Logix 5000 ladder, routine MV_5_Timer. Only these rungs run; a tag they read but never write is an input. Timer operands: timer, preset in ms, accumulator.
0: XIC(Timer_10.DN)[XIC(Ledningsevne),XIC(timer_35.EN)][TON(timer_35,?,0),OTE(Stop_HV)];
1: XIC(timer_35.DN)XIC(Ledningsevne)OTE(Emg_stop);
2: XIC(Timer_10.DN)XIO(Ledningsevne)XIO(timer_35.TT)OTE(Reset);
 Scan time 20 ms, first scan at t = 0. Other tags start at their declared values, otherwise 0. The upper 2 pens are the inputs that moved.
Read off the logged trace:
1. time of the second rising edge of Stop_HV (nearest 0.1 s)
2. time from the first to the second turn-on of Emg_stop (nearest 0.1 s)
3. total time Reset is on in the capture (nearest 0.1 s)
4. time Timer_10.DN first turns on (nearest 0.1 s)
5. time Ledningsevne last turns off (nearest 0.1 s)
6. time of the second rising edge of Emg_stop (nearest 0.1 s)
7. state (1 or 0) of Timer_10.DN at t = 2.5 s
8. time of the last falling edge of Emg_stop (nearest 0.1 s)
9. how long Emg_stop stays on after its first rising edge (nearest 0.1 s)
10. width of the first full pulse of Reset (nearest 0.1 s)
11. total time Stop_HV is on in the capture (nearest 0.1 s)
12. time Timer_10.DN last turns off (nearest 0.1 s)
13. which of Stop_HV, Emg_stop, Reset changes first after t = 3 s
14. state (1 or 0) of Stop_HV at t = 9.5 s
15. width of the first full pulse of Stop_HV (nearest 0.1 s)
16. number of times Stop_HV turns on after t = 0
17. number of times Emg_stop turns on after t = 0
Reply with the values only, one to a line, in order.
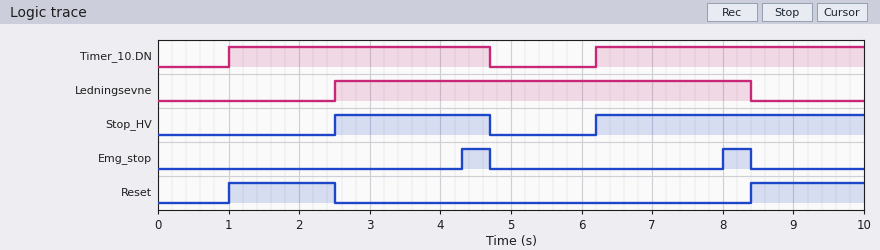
6.2 s
3.7 s
3.1 s
1.0 s
8.4 s
8.0 s
1
8.4 s
0.4 s
1.5 s
6.0 s
4.7 s
Emg_stop
1
2.2 s
2
2
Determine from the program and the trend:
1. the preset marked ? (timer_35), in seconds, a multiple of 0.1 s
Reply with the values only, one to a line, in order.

1.8 s
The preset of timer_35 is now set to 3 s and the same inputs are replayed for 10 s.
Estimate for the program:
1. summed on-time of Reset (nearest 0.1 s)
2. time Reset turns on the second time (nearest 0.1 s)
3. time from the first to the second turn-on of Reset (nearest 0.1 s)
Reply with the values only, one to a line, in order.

2.3 s
9.2 s
8.2 s
